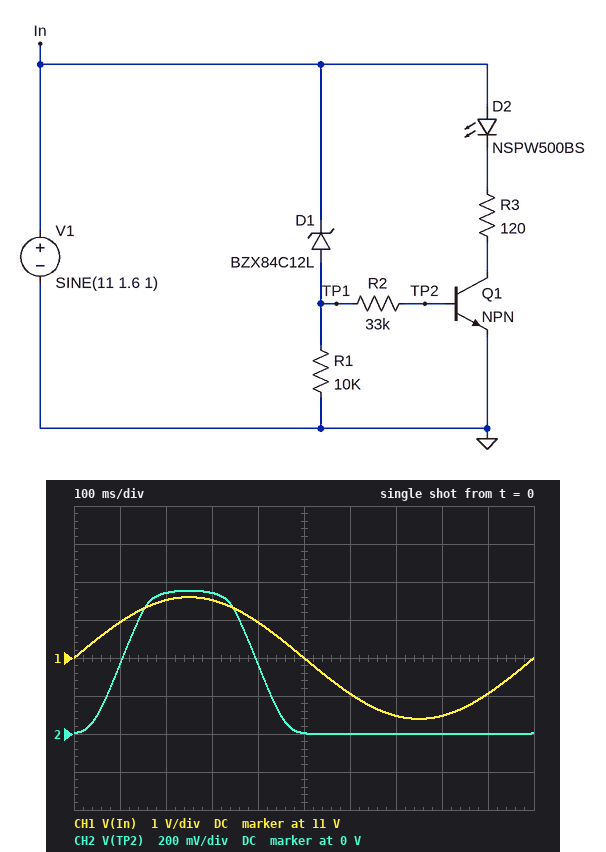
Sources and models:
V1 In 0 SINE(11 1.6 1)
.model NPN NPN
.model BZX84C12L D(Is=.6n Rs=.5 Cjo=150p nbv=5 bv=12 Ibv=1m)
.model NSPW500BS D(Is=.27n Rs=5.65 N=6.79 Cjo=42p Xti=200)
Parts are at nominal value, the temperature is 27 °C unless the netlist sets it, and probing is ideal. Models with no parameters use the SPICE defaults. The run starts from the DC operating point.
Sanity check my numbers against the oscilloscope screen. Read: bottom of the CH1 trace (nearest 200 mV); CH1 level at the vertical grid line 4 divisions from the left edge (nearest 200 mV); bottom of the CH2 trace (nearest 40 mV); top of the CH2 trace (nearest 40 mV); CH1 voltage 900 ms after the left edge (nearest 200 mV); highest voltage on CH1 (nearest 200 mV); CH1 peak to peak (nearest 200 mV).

9.4 V
12.0 V
0 V
760 mV
10.0 V
12.6 V
3.2 V
